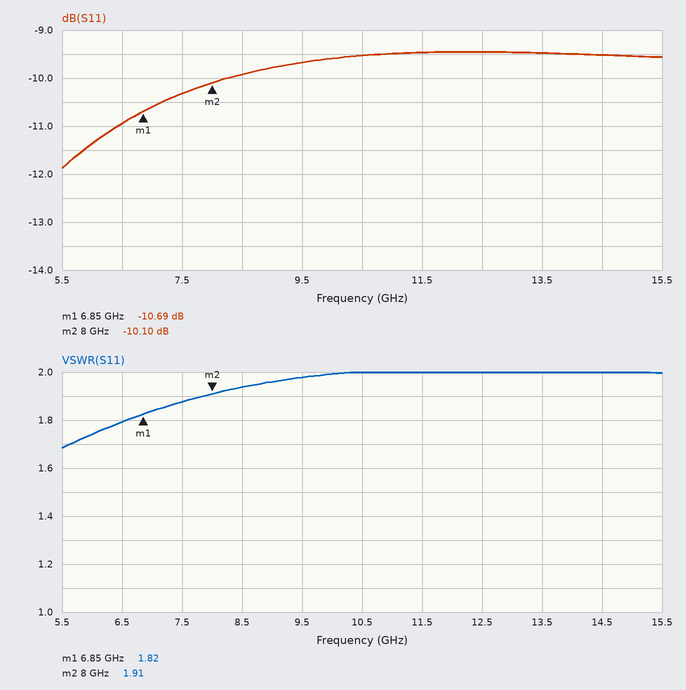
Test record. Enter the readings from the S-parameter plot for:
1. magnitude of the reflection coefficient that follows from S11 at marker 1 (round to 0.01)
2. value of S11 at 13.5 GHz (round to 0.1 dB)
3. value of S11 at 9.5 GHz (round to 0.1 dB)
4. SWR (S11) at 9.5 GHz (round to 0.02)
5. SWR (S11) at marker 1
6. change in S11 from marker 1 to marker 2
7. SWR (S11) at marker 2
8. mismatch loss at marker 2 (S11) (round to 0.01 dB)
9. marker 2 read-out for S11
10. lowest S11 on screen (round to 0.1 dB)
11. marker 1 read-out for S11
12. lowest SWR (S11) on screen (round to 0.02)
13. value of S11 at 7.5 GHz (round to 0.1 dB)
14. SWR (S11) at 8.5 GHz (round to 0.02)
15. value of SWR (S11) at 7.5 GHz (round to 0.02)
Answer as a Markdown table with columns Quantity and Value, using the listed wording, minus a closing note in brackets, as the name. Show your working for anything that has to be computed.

| Quantity | Value |
|---|---|
| magnitude of the reflection coefficient that follows from S11 at marker 1 | 10^(-10.69/20) ≈ 0.29 |
| value of S11 at 13.5 GHz | -9.5 dB |
| value of S11 at 9.5 GHz | -9.7 dB |
| SWR (S11) at 9.5 GHz | 1.98 |
| SWR (S11) at marker 1 | 1.82 |
| change in S11 from marker 1 to marker 2 | -10.1 − (-10.69) = 0.59 dB |
| SWR (S11) at marker 2 | 1.91 |
| mismatch loss at marker 2 (S11) | −10 log10(1 − 10^(-10.1/10)) ≈ 0.45 dB |
| marker 2 read-out for S11 | -10.10 dB |
| lowest S11 on screen | -11.9 dB |
| marker 1 read-out for S11 | -10.69 dB |
| lowest SWR (S11) on screen | 1.68 |
| value of S11 at 7.5 GHz | -10.3 dB |
| SWR (S11) at 8.5 GHz | 1.94 |
| value of SWR (S11) at 7.5 GHz | 1.88 |
